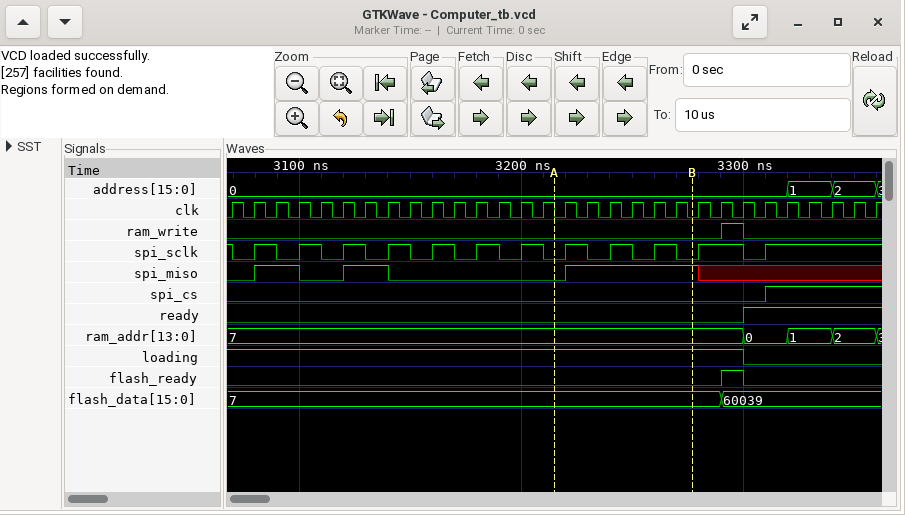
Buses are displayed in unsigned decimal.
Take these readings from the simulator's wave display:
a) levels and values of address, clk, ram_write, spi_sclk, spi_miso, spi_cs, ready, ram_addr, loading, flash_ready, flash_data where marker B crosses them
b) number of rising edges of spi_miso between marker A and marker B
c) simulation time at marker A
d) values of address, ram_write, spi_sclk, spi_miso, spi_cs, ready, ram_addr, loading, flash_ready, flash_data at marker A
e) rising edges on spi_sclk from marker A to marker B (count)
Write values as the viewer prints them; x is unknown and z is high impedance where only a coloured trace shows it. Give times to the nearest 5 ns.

address=0, clk=0, ram_write=0, spi_sclk=0, spi_miso=1, spi_cs=0, ready=0, ram_addr=7, loading=1, flash_ready=0, flash_data=7
1
3215 ns
address=0, ram_write=0, spi_sclk=0, spi_miso=0, spi_cs=0, ready=0, ram_addr=7, loading=1, flash_ready=0, flash_data=7
3
